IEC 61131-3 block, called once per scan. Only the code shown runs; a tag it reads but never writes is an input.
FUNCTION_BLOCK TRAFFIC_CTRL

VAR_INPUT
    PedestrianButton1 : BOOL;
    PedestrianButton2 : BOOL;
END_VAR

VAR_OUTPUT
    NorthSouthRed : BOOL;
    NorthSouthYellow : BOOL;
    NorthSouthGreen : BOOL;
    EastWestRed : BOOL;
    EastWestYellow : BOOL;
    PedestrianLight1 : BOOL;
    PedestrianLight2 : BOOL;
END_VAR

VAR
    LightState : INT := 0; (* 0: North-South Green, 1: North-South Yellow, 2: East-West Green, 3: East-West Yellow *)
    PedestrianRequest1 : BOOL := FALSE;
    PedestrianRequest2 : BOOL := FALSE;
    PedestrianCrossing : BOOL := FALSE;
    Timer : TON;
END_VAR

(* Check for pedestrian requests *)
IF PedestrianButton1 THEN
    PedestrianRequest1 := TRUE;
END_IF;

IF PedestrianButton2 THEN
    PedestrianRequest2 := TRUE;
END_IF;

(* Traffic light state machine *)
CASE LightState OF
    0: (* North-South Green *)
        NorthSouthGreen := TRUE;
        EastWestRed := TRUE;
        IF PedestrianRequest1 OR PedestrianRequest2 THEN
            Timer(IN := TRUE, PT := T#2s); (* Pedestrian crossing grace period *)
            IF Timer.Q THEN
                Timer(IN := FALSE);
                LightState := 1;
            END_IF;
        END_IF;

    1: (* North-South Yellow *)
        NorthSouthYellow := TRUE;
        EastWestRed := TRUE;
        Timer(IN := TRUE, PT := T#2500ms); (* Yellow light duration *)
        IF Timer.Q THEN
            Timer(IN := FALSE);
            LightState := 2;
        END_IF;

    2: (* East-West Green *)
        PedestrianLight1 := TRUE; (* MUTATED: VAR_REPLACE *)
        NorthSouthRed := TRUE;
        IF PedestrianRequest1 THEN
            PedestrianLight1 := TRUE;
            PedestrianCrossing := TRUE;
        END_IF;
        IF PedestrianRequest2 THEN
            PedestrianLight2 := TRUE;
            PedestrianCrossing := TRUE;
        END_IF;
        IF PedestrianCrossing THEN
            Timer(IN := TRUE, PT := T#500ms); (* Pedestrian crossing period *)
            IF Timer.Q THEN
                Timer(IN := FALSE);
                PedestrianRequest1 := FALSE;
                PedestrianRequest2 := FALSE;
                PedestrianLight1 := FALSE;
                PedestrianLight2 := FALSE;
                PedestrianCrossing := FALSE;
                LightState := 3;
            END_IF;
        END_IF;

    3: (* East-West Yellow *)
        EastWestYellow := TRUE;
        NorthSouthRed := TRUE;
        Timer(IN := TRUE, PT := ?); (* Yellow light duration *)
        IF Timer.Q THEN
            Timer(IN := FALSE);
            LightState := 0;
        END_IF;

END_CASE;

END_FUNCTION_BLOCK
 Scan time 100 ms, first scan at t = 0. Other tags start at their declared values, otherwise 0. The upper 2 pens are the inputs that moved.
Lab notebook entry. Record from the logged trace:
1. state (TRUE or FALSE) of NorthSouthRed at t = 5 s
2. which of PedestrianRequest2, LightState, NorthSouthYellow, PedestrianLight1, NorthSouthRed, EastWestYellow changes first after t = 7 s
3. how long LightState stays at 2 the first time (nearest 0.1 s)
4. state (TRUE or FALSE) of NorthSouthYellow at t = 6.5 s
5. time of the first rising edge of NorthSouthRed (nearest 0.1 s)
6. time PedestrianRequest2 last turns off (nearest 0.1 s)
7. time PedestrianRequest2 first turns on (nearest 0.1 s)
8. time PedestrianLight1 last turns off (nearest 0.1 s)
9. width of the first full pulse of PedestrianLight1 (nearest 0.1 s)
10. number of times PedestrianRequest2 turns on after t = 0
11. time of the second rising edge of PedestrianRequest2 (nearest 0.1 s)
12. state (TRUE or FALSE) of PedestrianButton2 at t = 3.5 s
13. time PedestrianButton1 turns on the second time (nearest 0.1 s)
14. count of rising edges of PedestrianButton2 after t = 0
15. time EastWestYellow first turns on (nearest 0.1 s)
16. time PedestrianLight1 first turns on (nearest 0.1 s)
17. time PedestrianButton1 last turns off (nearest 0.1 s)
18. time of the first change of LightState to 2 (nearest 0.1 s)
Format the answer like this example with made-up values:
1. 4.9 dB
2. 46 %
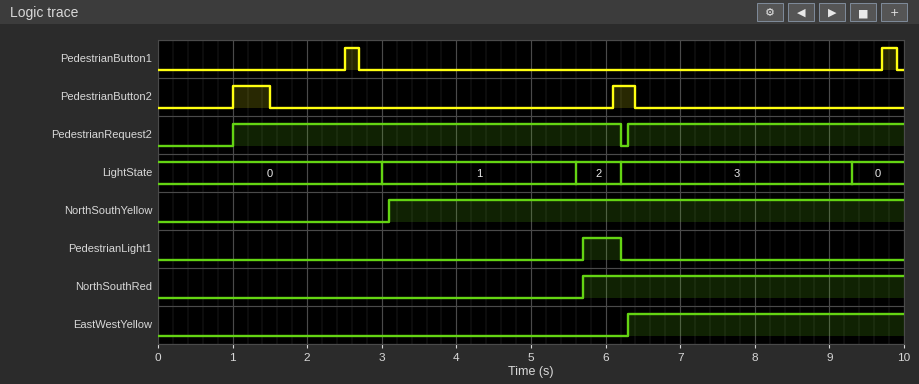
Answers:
1. FALSE
2. LightState
3. 0.6 s
4. TRUE
5. 5.7 s
6. 6.2 s
7. 1.0 s
8. 6.2 s
9. 0.5 s
10. 2
11. 6.3 s
12. FALSE
13. 9.7 s
14. 2
15. 6.3 s
16. 5.7 s
17. 9.9 s
18. 5.6 s
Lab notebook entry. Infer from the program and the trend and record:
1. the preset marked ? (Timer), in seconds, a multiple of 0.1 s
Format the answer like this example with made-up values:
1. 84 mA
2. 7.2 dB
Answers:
1. 3.0 s
